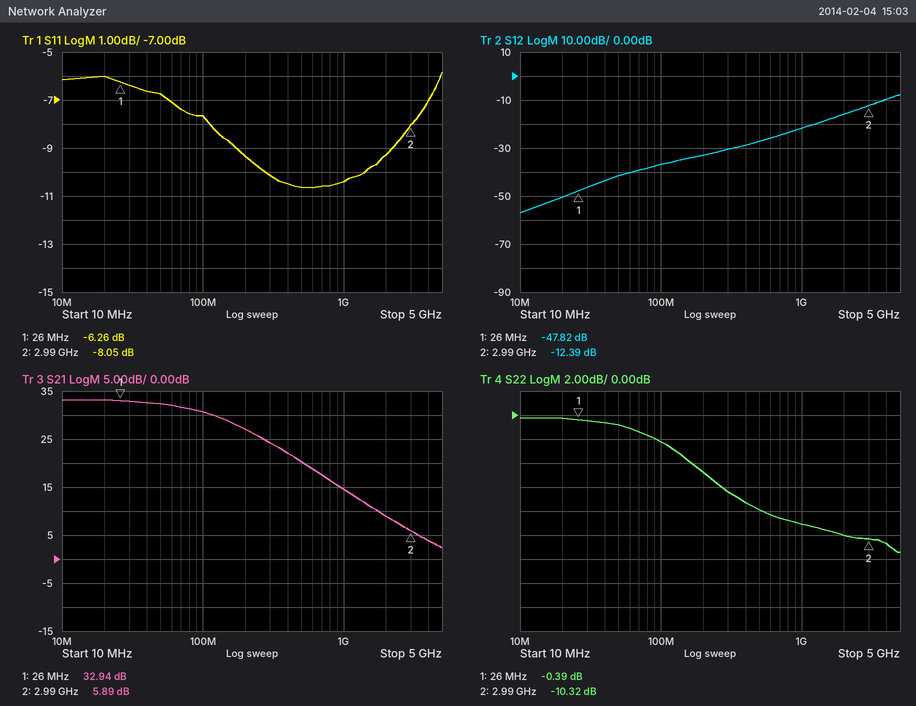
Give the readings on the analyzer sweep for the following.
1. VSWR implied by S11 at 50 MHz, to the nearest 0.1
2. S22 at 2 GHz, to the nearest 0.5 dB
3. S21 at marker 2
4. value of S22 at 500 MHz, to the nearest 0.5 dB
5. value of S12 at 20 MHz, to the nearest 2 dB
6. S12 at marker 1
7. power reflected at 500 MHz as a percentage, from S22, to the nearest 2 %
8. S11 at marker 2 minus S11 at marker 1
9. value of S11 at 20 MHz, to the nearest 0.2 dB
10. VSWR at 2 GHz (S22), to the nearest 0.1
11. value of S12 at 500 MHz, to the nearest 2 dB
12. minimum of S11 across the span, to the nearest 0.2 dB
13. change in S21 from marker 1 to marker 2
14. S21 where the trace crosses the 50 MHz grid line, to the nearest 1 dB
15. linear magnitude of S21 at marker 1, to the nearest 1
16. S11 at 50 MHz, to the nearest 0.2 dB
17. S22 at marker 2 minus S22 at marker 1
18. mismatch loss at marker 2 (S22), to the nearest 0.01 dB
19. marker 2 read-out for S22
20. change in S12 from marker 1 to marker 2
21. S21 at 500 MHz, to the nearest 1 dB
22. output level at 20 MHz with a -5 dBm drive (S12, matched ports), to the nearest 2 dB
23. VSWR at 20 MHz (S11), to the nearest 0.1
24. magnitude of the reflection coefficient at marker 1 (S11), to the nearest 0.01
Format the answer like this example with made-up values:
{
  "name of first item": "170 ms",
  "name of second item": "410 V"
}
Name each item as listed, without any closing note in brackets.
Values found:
{
  "VSWR implied by S11 at 50 MHz, to the nearest 0.1": "2.7",
  "S22 at 2 GHz, to the nearest 0.5 dB": "-10.0 dB",
  "S21 at marker 2": "5.89 dB",
  "value of S22 at 500 MHz, to the nearest 0.5 dB": "-8.0 dB",
  "value of S12 at 20 MHz, to the nearest 2 dB": "-50 dB",
  "S12 at marker 1": "-47.82 dB",
  "power reflected at 500 MHz as a percentage, from S22, to the nearest 2 %": "16 %",
  "S11 at marker 2 minus S11 at marker 1": "-1.79 dB",
  "value of S11 at 20 MHz, to the nearest 0.2 dB": "-6.0 dB",
  "VSWR at 2 GHz (S22), to the nearest 0.1": "1.9",
  "value of S12 at 500 MHz, to the nearest 2 dB": "-28 dB",
  "minimum of S11 across the span, to the nearest 0.2 dB": "-10.6 dB",
  "change in S21 from marker 1 to marker 2": "-27.05 dB",
  "S21 where the trace crosses the 50 MHz grid line, to the nearest 1 dB": "32 dB",
  "linear magnitude of S21 at marker 1, to the nearest 1": "44",
  "S11 at 50 MHz, to the nearest 0.2 dB": "-6.8 dB",
  "S22 at marker 2 minus S22 at marker 1": "-9.93 dB",
  "mismatch loss at marker 2 (S22), to the nearest 0.01 dB": "0.42 dB",
  "marker 2 read-out for S22": "-10.32 dB",
  "change in S12 from marker 1 to marker 2": "35.43 dB",
  "S21 at 500 MHz, to the nearest 1 dB": "20 dB",
  "output level at 20 MHz with a -5 dBm drive (S12, matched ports), to the nearest 2 dB": "-56 dBm",
  "VSWR at 20 MHz (S11), to the nearest 0.1": "3.0",
  "magnitude of the reflection coefficient at marker 1 (S11), to the nearest 0.01": "0.49"
}
